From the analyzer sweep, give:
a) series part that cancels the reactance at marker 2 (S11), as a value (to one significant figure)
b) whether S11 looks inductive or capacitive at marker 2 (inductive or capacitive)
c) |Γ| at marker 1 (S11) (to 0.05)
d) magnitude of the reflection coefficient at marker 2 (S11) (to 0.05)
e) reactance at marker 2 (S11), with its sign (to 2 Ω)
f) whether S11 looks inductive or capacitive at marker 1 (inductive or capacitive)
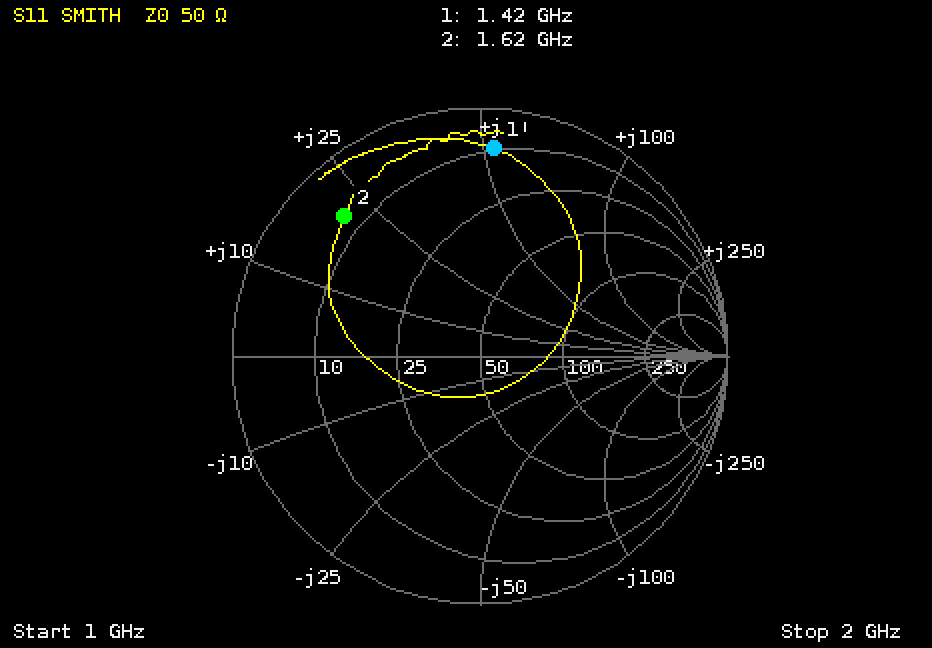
5 pF
inductive
0.85
0.80
+20 Ω
inductive
